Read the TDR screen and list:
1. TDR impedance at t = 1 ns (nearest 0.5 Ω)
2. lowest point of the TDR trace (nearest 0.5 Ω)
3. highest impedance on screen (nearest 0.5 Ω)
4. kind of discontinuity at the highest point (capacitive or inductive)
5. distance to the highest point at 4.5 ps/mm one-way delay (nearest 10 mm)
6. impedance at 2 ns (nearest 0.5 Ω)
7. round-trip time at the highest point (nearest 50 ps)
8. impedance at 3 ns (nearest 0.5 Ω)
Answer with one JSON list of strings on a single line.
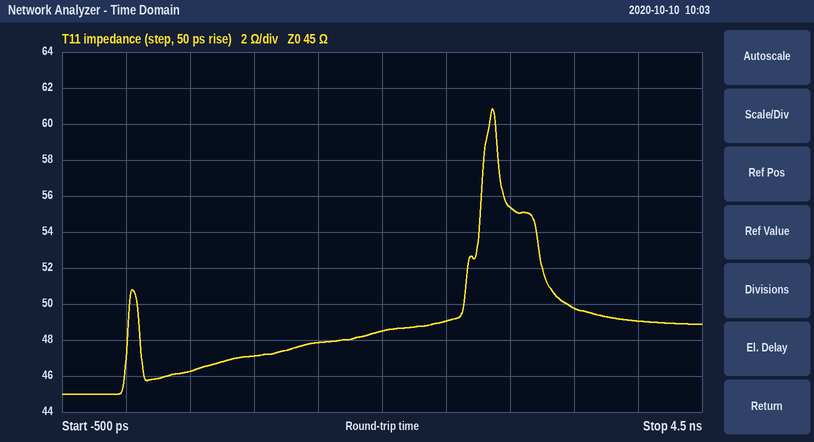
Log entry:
["47.0 Ω", "45.0 Ω", "61.0 Ω", "inductive", "320 mm", "48.5 Ω", "2.85 ns", "55.5 Ω"]
